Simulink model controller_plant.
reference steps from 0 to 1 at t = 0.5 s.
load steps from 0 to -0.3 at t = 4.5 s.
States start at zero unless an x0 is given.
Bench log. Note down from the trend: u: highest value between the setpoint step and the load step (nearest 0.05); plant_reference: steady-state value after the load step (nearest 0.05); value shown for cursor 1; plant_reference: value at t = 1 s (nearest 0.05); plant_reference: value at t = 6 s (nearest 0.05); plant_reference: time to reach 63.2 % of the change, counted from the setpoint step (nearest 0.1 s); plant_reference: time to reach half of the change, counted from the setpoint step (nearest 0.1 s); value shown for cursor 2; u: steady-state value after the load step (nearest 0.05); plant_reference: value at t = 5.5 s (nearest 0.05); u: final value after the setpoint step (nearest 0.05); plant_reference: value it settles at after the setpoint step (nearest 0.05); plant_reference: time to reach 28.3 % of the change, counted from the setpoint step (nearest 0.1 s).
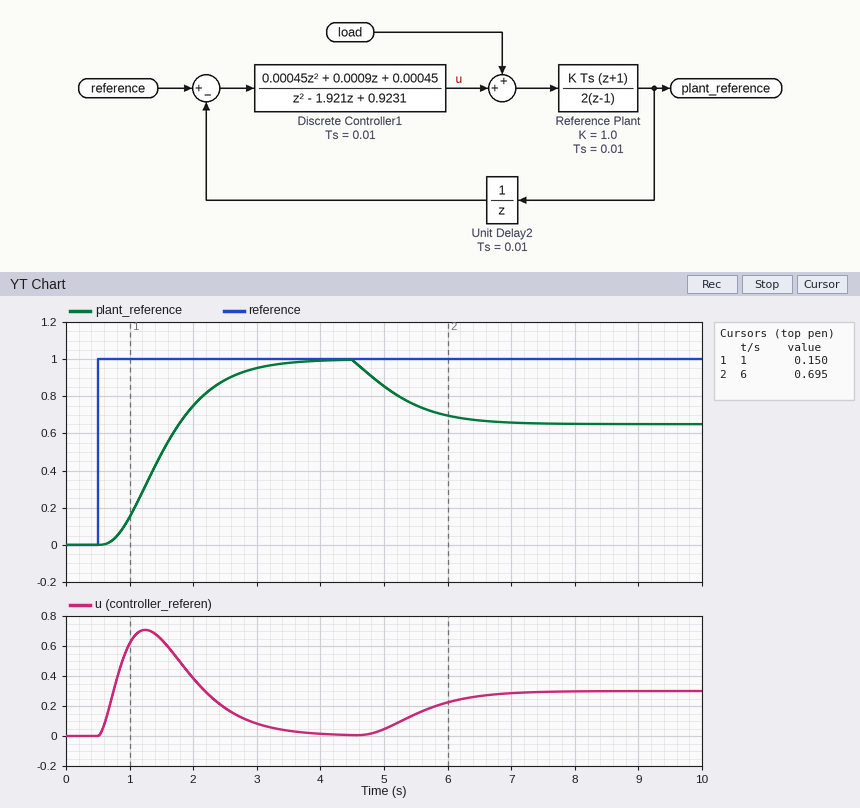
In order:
0.70
0.65
0.150
0.15
0.70
1.2 s
1.0 s
0.695
0.30
0.75
0.00
1.00
0.7 s
